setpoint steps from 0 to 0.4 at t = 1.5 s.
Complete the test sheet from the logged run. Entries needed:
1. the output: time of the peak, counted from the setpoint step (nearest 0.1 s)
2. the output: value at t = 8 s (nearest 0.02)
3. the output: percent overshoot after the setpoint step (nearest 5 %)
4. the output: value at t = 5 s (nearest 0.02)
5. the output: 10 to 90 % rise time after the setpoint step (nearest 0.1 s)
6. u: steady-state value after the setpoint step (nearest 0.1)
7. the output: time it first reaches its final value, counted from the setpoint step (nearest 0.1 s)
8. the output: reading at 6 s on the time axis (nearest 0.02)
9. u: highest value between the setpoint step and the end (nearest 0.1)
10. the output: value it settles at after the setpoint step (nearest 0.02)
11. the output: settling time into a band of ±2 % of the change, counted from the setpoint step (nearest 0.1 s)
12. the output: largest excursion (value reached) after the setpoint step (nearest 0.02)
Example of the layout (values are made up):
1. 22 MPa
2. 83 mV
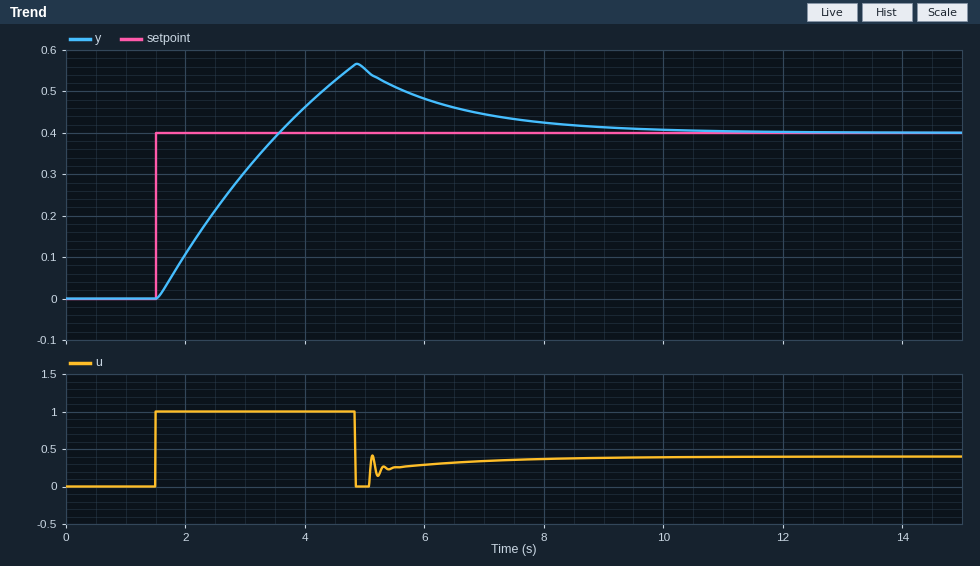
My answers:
1. 3.4 s
2. 0.42
3. 40 %
4. 0.56
5. 1.6 s
6. 0.4
7. 2.1 s
8. 0.48
9. 1.0
10. 0.40
11. 8.4 s
12. 0.56
